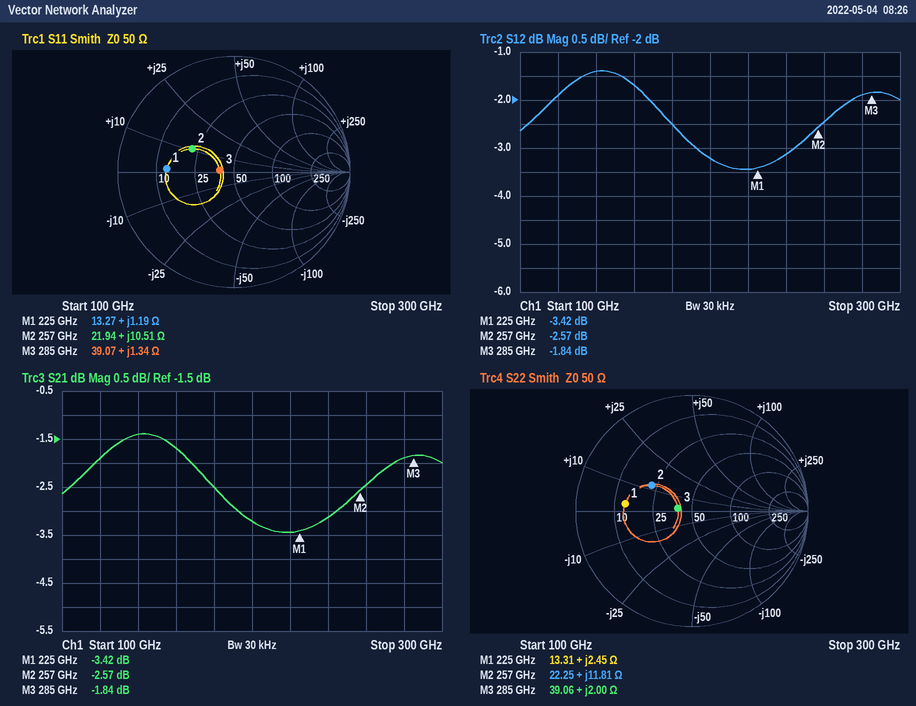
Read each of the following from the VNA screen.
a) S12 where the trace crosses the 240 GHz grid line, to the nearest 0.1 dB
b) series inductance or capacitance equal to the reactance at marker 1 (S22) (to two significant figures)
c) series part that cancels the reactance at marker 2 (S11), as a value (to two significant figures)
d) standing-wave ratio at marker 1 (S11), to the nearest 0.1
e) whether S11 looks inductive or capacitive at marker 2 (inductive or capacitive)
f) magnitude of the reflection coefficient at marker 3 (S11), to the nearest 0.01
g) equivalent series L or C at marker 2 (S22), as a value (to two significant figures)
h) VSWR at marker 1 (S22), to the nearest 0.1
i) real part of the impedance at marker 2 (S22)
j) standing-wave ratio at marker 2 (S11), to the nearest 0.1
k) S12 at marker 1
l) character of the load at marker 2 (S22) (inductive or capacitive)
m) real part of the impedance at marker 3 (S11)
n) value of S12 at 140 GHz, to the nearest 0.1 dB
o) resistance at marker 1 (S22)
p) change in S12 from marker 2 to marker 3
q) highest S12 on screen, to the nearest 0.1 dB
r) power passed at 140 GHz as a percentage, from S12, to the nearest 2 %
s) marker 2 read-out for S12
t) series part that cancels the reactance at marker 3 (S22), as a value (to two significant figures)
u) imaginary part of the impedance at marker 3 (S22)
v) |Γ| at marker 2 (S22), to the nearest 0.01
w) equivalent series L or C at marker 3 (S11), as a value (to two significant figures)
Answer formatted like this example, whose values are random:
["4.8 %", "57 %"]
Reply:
["-3.1 dB", "1.7 pH", "59 fF", "3.8", "inductive", "0.12", "7.3 pH", "3.8", "22.25 Ω", "2.4", "-3.42 dB", "inductive", "39.07 Ω", "-1.4 dB", "13.31 Ω", "0.73 dB", "-1.4 dB", "72 %", "-2.57 dB", "280 fF", "+2.00 Ω", "0.41", "750 fH"]
